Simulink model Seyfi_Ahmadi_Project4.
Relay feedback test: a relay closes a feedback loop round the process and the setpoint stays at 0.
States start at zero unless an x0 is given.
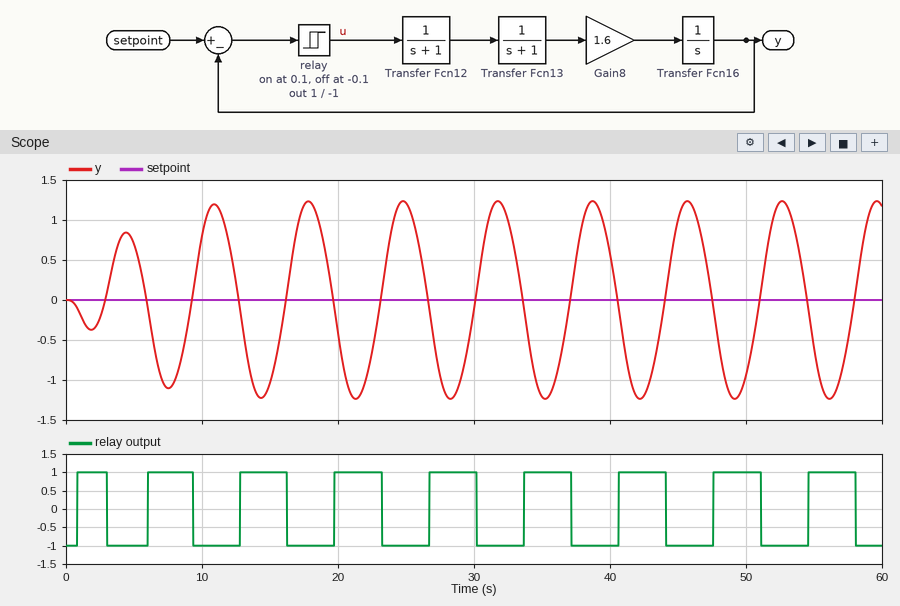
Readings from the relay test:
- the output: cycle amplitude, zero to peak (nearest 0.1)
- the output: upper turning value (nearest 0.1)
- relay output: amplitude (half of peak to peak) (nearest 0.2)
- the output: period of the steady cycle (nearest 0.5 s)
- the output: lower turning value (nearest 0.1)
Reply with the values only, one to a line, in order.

1.2
1.2
1.0
7.0 s
-1.2
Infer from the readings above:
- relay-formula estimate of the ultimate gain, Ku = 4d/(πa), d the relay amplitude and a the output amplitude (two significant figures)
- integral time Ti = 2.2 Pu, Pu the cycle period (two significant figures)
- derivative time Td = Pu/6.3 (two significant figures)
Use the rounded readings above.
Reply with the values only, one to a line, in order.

1.1
15 s
1.1 s
